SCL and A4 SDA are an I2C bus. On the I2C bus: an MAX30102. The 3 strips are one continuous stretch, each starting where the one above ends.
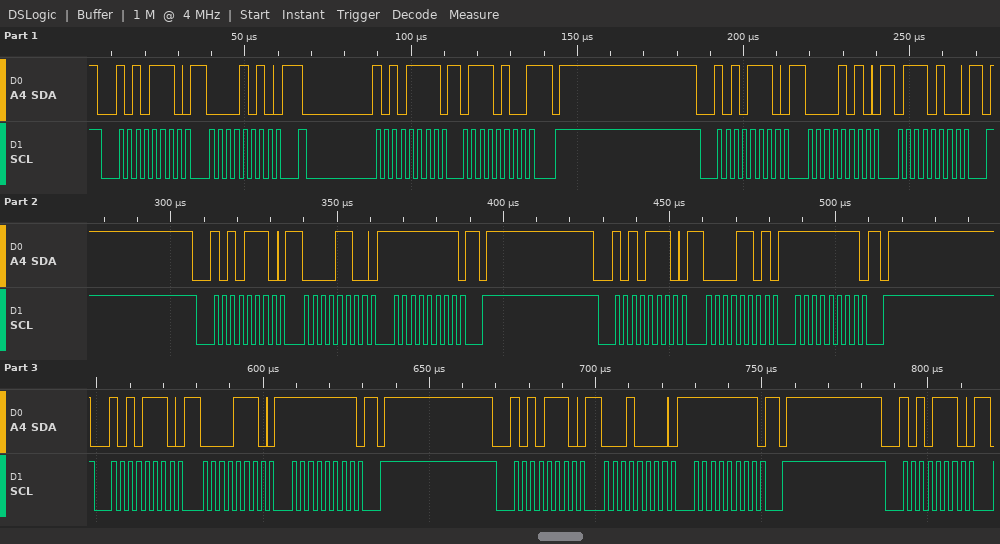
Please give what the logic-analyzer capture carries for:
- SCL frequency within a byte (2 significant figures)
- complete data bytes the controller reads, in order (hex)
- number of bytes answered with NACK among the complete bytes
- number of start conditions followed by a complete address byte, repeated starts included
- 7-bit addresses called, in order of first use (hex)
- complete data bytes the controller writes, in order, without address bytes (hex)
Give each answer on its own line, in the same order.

400 kHz
74
1
8
0x57
0A 0A 74 0C FF 0D FF 0E FF 10 FF
